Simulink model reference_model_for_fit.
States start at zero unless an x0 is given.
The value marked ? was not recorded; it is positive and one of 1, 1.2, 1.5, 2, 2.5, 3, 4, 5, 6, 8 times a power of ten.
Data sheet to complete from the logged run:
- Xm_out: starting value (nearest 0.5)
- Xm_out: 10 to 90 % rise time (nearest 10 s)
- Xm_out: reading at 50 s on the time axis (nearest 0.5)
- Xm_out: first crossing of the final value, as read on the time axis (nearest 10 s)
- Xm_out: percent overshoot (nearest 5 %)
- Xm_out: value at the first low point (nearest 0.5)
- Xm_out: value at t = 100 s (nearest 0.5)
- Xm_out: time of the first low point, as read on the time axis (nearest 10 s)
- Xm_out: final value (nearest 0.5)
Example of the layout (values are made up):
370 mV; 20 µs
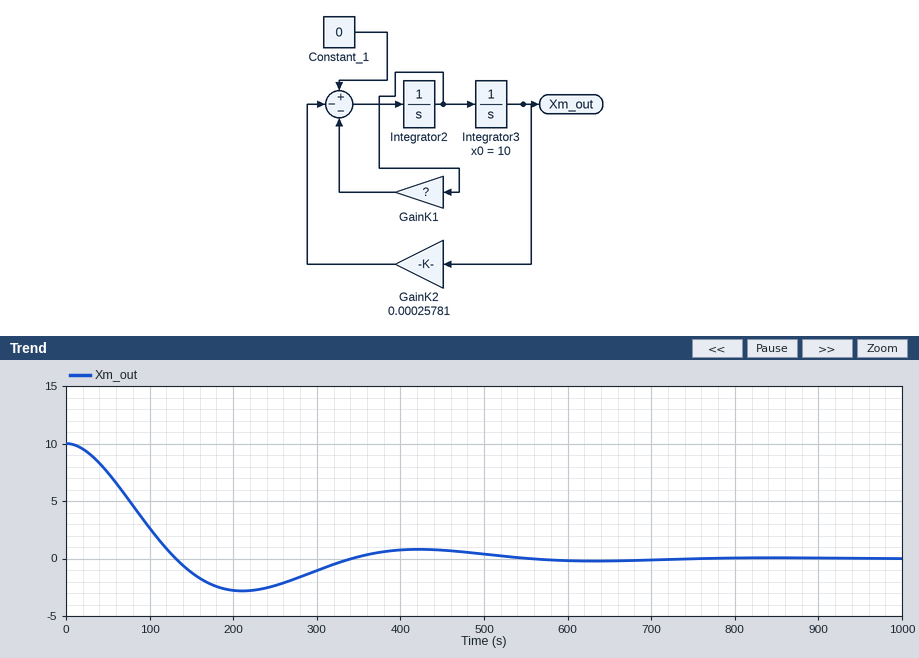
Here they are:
10.0; 90 s; 7.5; 130 s; 30 %; -3.0; 2.5; 210 s; 0.0
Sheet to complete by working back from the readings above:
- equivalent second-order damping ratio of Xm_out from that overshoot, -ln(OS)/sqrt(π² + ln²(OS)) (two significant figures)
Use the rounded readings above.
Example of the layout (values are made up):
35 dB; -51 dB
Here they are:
0.36
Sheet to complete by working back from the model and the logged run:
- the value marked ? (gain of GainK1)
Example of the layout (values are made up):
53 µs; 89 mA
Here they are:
0.012
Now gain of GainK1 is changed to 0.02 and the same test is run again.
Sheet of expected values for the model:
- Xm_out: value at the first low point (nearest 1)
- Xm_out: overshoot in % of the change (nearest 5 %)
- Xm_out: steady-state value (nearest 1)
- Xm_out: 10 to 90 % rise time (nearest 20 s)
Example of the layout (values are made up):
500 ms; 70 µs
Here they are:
-1; 10 %; 0; 120 s
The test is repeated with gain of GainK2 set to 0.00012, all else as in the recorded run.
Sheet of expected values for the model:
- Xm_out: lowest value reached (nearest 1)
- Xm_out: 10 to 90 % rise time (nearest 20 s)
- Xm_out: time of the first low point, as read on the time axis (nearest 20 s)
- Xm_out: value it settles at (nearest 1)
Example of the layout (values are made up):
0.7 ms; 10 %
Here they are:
-1; 160 s; 340 s; 0
